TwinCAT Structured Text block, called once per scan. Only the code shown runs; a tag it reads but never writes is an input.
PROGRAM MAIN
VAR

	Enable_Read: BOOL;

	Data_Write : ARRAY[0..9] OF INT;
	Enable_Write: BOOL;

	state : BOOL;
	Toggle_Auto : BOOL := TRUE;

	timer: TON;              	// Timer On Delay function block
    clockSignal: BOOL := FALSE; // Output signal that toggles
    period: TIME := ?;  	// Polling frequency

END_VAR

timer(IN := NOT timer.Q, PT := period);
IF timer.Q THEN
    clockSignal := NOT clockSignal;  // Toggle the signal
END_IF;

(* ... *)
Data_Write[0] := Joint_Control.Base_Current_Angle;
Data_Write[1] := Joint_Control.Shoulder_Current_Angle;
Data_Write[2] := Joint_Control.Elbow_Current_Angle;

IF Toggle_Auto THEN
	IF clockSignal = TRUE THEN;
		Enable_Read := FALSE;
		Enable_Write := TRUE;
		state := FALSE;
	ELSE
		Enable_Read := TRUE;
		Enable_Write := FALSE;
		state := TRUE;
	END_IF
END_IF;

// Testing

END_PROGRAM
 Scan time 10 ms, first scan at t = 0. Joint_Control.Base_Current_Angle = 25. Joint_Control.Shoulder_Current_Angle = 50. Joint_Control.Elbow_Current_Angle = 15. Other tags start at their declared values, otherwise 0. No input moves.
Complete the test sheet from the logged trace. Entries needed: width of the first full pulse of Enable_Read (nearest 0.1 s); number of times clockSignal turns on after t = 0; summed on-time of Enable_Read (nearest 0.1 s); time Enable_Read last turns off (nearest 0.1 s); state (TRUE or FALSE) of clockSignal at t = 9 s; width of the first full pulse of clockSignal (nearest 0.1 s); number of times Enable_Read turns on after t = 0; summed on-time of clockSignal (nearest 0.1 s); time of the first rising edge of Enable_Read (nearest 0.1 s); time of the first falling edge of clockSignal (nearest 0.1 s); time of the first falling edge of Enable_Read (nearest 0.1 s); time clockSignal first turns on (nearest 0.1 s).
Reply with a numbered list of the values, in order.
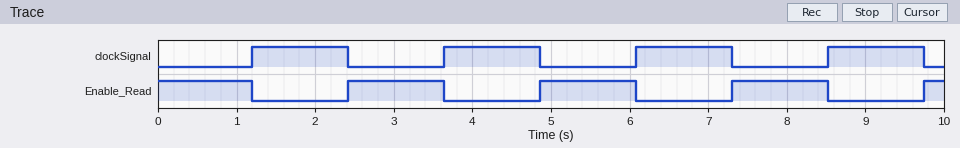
1. 1.2 s
2. 4
3. 5.1 s
4. 8.5 s
5. TRUE
6. 1.2 s
7. 4
8. 4.9 s
9. 2.4 s
10. 2.4 s
11. 1.2 s
12. 1.2 s
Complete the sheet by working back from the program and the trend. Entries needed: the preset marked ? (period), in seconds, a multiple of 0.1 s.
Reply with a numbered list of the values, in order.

1. 1.2 s
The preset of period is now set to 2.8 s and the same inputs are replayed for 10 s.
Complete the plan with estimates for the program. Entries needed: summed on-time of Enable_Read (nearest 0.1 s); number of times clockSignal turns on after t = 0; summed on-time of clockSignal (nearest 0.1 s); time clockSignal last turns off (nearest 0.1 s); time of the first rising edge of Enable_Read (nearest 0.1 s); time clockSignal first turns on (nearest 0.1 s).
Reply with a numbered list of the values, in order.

1. 5.6 s
2. 2
3. 4.4 s
4. 5.6 s
5. 5.6 s
6. 2.8 s
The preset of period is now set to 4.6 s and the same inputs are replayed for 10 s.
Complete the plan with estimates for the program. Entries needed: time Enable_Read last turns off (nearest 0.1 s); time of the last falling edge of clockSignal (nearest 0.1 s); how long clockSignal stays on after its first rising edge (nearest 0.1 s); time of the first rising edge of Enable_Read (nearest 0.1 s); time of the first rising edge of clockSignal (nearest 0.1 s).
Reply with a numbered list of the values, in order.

1. 4.6 s
2. 9.2 s
3. 4.6 s
4. 9.2 s
5. 4.6 s
